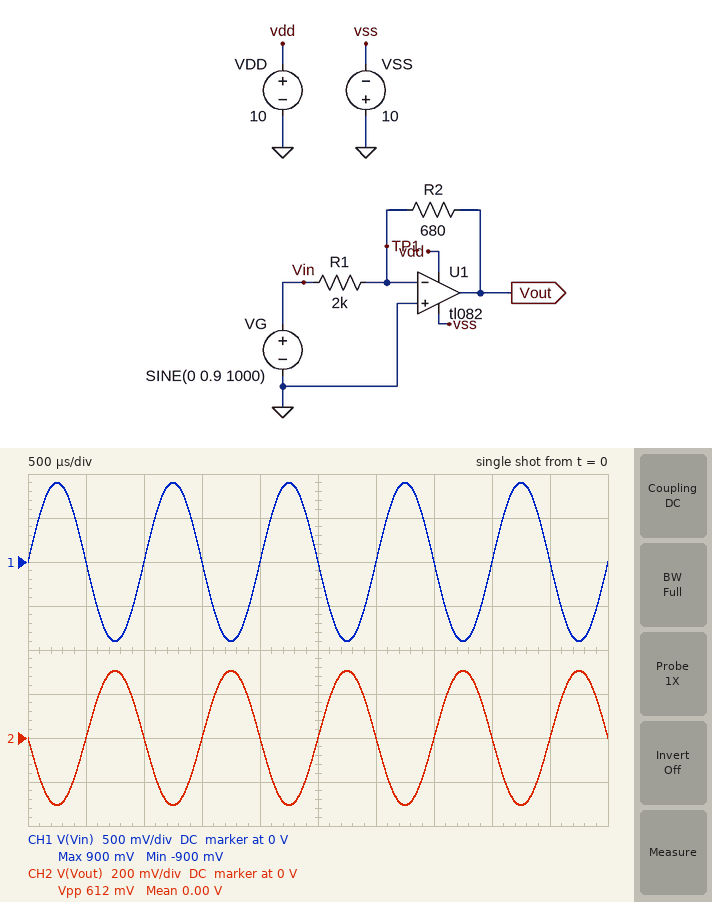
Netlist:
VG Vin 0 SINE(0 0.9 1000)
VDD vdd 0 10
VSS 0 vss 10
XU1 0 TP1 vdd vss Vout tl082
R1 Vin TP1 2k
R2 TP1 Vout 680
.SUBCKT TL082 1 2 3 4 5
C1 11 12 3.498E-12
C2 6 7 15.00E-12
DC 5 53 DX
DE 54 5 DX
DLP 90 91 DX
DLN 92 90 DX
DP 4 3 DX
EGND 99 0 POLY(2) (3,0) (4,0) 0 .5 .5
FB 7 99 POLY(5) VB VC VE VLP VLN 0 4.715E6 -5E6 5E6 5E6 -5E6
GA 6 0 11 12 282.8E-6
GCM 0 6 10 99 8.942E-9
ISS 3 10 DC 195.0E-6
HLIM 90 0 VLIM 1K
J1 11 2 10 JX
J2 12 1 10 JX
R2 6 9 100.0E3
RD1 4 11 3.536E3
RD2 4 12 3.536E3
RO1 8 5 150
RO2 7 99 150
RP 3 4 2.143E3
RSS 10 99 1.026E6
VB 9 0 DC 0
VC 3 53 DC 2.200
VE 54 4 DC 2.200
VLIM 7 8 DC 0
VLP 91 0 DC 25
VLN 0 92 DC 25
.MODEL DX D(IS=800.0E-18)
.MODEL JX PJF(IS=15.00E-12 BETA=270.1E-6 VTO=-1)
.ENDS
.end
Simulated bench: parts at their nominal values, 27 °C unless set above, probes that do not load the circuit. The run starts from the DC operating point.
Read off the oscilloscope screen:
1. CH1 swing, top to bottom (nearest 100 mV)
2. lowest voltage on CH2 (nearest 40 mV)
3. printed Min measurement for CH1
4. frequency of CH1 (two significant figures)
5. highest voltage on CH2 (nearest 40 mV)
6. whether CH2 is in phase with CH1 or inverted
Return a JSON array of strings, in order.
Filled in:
["1.8 V", "-320 mV", "-900 mV", "1.0 kHz", "320 mV", "inverted"]
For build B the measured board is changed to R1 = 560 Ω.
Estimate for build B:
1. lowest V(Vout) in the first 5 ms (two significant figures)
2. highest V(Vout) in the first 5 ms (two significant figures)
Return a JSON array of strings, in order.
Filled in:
["-1.1 V", "1.1 V"]
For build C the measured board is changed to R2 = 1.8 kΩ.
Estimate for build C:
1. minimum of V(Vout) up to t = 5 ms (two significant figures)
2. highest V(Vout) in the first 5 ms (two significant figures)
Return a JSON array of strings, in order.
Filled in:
["-810 mV", "810 mV"]
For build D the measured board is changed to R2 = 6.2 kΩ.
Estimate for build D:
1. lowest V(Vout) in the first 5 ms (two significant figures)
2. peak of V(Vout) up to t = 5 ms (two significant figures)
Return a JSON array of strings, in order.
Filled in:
["-2.8 V", "2.8 V"]
